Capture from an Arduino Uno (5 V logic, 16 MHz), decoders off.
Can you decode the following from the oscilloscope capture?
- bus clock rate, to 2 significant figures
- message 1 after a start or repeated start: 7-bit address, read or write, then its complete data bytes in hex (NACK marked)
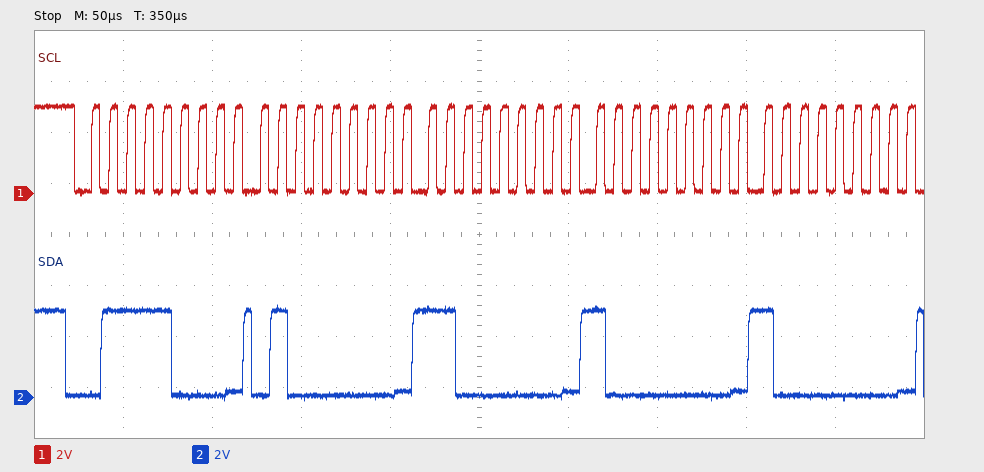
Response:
100 kHz
0x3C write: 40 C0 80 80
